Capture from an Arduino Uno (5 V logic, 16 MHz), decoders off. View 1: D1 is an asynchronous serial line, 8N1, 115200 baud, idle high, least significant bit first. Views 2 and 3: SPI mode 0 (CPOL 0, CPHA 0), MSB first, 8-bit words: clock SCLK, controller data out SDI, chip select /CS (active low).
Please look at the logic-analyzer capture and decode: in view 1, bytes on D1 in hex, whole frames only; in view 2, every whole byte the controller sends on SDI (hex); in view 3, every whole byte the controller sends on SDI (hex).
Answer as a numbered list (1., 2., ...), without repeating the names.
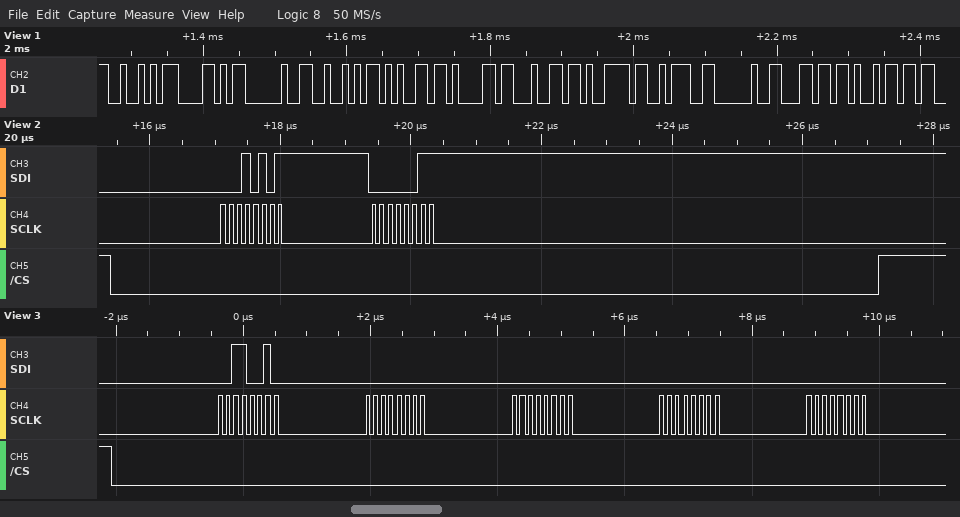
1. 0x52 0x58 0x20 0x52 0x65 0x61 0x64 0x79 0x3A 0x20 0x6C 0x69
2. 15 03
3. 32 00 00 00 00
